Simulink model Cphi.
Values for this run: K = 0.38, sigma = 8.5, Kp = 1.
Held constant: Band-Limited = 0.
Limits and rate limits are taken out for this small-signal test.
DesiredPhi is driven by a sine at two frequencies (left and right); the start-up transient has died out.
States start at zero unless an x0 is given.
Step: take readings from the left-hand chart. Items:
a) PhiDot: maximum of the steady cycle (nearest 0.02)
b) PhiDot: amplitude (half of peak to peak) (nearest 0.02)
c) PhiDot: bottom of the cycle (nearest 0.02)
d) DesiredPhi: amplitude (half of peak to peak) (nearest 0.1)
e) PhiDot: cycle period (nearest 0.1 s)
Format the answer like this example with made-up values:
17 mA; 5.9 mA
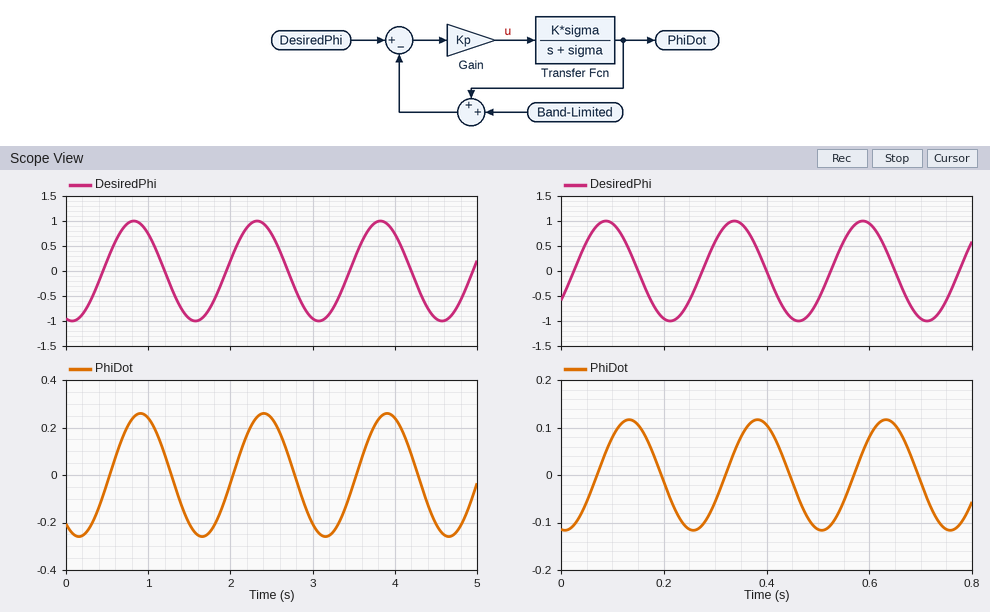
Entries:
0.26; 0.26; -0.26; 1.0; 1.5 s
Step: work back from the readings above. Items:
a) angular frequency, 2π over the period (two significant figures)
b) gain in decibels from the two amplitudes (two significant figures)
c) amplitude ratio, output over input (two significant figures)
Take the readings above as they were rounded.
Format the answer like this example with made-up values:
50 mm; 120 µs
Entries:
4.2 rad/s; -12 dB; 0.26
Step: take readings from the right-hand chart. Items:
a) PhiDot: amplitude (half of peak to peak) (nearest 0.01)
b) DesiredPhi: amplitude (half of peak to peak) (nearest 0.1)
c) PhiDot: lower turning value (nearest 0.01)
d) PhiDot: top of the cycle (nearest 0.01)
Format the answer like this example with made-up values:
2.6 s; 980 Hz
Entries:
0.12; 1.0; -0.12; 0.12
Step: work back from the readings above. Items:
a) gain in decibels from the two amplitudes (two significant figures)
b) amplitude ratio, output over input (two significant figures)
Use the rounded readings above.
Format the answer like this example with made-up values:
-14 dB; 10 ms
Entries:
-18 dB; 0.12
